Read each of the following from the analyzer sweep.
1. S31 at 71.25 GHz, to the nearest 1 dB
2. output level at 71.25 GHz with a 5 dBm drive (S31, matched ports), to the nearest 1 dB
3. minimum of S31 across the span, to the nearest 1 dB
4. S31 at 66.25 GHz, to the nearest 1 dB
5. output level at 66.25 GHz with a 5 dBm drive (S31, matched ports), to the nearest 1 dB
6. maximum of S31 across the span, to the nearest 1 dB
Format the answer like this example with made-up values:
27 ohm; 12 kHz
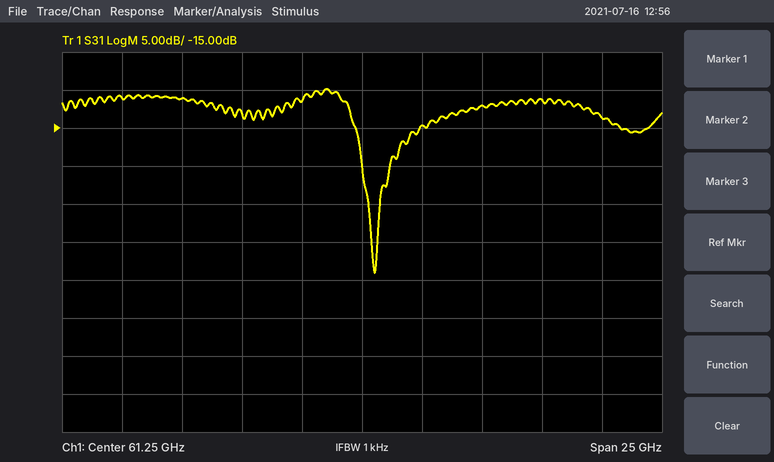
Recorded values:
-14 dB; -9 dBm; -34 dB; -12 dB; -7 dBm; -10 dB
